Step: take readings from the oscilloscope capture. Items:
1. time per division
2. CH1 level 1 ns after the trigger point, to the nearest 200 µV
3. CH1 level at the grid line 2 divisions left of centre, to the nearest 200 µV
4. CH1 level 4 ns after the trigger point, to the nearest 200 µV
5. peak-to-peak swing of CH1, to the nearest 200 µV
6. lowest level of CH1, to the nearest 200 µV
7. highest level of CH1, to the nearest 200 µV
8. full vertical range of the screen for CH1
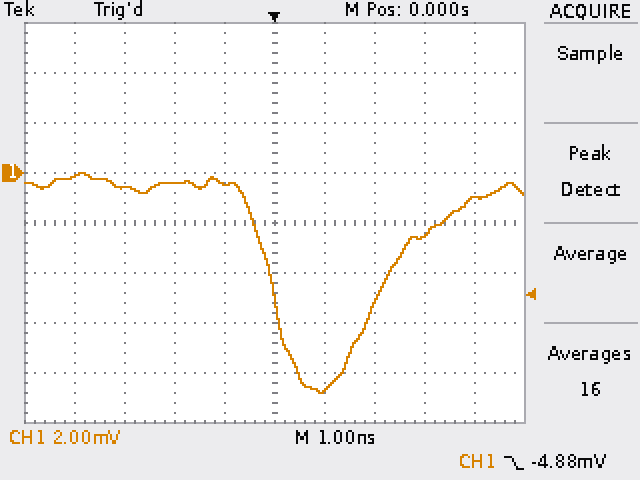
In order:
1 ns
-8.6 mV
-400 µV
-1.0 mV
8.8 mV
-8.8 mV
0.0 mV
16 mV
